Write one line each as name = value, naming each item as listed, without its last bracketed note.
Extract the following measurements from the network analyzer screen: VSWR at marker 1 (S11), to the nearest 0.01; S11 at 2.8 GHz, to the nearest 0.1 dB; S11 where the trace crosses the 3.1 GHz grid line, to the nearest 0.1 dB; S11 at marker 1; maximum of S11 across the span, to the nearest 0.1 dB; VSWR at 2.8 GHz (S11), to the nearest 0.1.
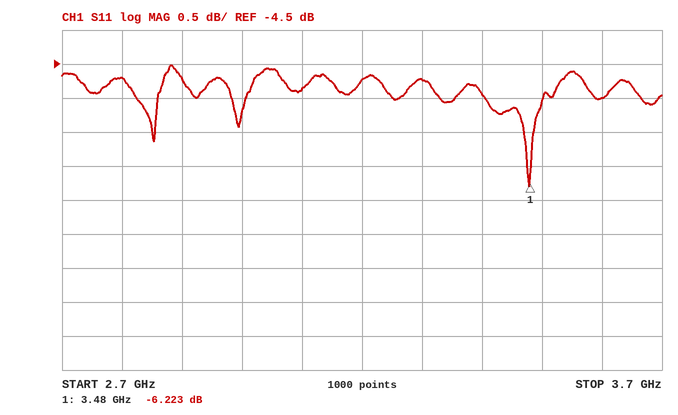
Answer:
VSWR at marker 1 (S11), to the nearest 0.01 = 2.91
S11 at 2.8 GHz, to the nearest 0.1 dB = -4.7 dB
S11 where the trace crosses the 3.1 GHz grid line, to the nearest 0.1 dB = -4.9 dB
S11 at marker 1 = -6.223 dB
maximum of S11 across the span, to the nearest 0.1 dB = -4.5 dB
VSWR at 2.8 GHz (S11), to the nearest 0.1 = 3.8
